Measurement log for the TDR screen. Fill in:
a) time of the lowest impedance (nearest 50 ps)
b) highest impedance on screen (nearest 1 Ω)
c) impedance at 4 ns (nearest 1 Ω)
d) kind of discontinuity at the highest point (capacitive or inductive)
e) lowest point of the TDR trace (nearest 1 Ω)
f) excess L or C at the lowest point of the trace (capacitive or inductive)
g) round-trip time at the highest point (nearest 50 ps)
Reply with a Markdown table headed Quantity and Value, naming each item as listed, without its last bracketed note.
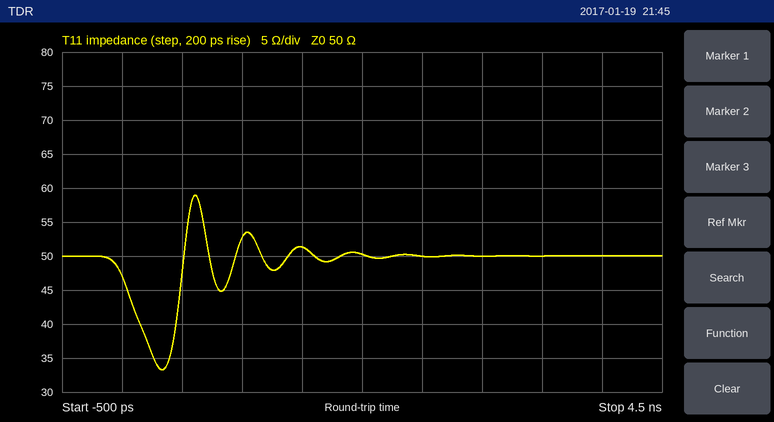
| Quantity | Value |
|---|---|
| time of the lowest impedance | 350 ps |
| highest impedance on screen | 59 Ω |
| impedance at 4 ns | 50 Ω |
| kind of discontinuity at the highest point | inductive |
| lowest point of the TDR trace | 33 Ω |
| excess L or C at the lowest point of the trace | capacitive |
| round-trip time at the highest point | 600 ps |
